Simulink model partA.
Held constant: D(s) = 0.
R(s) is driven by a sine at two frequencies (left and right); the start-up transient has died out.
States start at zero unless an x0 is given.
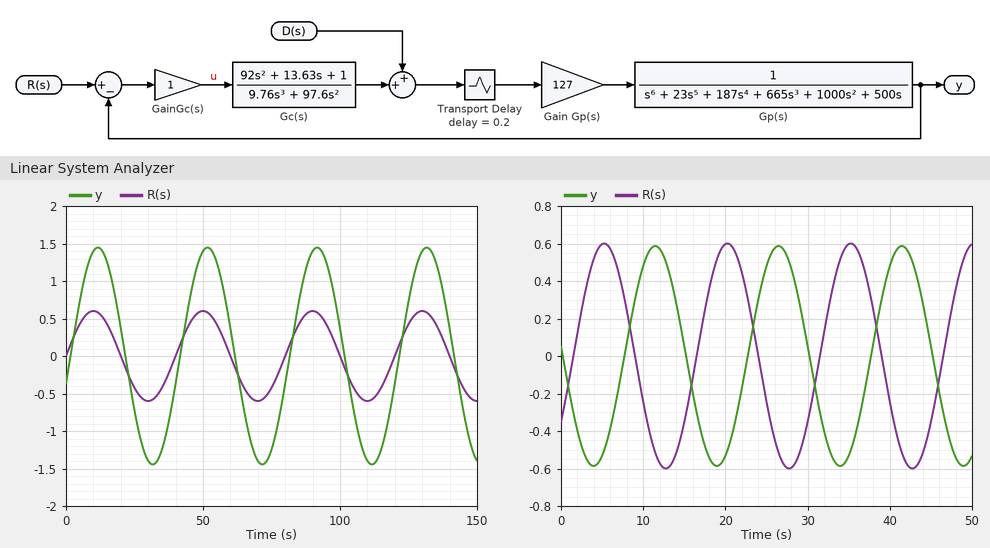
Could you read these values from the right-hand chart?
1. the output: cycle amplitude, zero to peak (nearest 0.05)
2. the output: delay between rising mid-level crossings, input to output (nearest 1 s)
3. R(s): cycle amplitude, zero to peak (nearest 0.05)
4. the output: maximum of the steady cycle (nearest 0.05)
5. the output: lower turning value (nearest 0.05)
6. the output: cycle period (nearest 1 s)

0.60
6 s
0.60
0.60
-0.60
15 s
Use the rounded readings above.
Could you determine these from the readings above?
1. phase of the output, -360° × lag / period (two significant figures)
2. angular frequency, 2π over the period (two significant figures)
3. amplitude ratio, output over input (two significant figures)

-140°
0.42 rad/s
1.0
